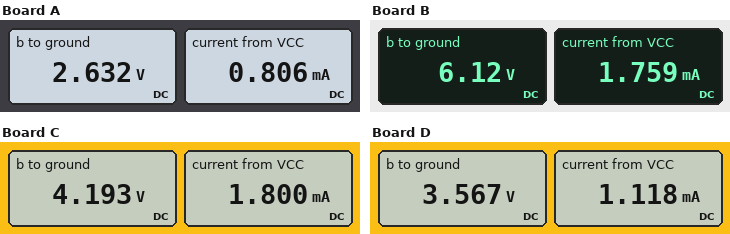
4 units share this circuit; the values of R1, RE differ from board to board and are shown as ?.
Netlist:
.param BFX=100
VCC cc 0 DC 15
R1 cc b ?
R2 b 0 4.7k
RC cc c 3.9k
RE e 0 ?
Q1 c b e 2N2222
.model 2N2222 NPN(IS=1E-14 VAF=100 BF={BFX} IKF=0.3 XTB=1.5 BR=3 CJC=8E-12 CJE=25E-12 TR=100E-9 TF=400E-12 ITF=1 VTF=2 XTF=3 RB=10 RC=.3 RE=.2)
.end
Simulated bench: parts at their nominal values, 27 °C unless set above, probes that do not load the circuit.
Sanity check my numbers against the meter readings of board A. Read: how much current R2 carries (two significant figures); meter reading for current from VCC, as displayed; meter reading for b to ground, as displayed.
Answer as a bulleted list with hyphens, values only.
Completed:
- 560 µA
- 0.806 mA
- 2.632 V
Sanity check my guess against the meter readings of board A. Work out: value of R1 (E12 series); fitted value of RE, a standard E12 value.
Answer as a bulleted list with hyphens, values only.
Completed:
- 22 kΩ
- 8.2 kΩ
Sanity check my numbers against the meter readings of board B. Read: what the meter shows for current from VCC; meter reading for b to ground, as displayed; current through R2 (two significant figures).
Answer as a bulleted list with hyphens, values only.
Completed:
- 1.759 mA
- 6.12 V
- 1.3 mA
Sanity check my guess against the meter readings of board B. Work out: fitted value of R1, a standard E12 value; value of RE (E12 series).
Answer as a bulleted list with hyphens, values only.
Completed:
- 6.8 kΩ
- 12 kΩ
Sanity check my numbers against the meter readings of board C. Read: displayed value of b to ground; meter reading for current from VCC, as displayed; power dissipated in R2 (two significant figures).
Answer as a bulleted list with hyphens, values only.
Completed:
- 4.193 V
- 1.800 mA
- 3.7 mW
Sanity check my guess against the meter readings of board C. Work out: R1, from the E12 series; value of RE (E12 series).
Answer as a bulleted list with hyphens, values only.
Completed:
- 12 kΩ
- 3.9 kΩ
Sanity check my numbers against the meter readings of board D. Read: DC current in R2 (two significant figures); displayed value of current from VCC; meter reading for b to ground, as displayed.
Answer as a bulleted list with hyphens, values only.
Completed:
- 760 µA
- 1.118 mA
- 3.567 V
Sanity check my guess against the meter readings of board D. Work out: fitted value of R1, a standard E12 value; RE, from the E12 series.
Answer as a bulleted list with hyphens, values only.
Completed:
- 15 kΩ
- 8.2 kΩ
